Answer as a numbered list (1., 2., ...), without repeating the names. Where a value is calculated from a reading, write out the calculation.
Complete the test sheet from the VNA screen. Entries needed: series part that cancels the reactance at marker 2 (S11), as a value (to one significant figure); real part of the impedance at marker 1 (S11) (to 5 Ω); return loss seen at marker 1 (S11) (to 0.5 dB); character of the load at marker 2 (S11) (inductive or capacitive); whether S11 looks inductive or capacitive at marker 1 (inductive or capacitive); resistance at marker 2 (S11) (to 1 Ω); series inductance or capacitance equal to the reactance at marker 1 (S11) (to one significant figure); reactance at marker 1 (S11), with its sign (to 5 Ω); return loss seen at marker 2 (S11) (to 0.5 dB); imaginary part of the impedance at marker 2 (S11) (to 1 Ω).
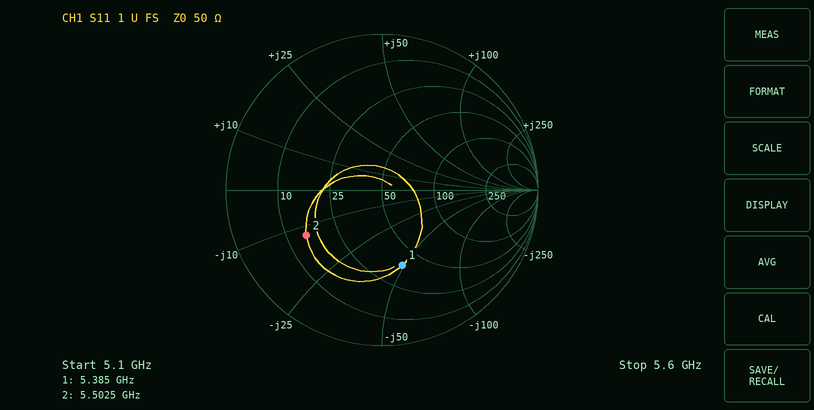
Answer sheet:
1. L = 13 Ω/(2π × 5.5025 GHz) ≈ 376 pH, so 400 pH to one significant figure
2. 40 Ω
3. 6.0 dB
4. capacitive
5. capacitive
6. 15 Ω
7. C = 1/(2π × 5.385 GHz × 50 Ω) ≈ 591 fF, so 600 fF to one significant figure
8. -50 Ω
9. 5.0 dB
10. -13 Ω
